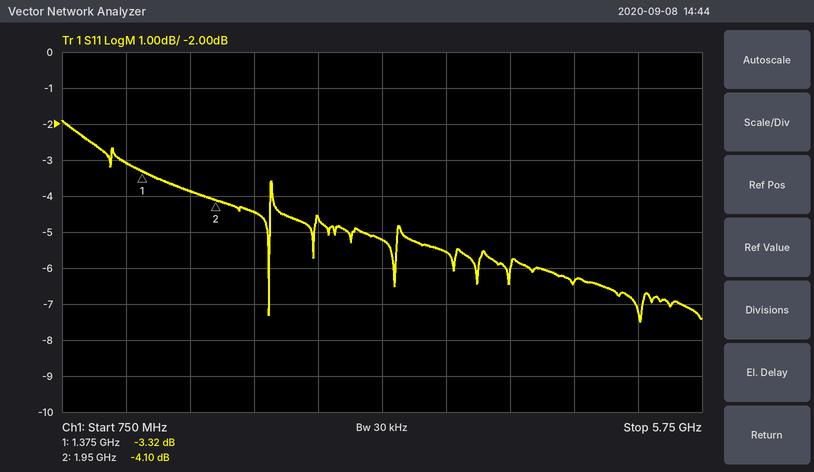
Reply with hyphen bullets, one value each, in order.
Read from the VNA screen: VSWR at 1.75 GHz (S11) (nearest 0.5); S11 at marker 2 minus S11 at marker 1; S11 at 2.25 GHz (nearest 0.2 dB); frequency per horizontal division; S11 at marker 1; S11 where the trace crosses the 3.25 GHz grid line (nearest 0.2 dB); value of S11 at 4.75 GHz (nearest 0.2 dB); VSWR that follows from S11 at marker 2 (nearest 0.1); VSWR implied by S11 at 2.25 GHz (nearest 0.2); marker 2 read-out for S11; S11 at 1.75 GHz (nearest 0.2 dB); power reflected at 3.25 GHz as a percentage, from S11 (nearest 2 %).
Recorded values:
- 4.5
- -0.78 dB
- -4.4 dB
- 500 MHz
- -3.32 dB
- -5.2 dB
- -6.4 dB
- 4.3
- 4.0
- -4.10 dB
- -3.8 dB
- 30 %
